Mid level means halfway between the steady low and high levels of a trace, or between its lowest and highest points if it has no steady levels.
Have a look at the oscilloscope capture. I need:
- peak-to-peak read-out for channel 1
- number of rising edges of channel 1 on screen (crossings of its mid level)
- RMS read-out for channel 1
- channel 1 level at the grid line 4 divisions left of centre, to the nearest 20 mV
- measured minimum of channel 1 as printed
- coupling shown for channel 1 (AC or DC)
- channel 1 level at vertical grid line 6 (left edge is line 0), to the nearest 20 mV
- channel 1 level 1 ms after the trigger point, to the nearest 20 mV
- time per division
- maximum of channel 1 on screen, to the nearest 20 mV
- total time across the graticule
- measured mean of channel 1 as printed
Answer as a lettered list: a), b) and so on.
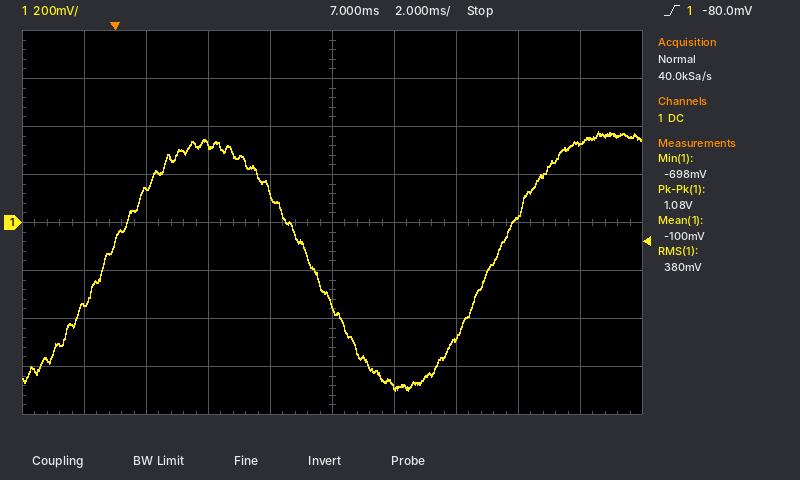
a) 1.08 V
b) 2
c) 380 mV
d) -340 mV
e) -698 mV
f) DC
g) -680 mV
h) 140 mV
i) 2 ms
j) 380 mV
k) 20 ms
l) -100 mV
